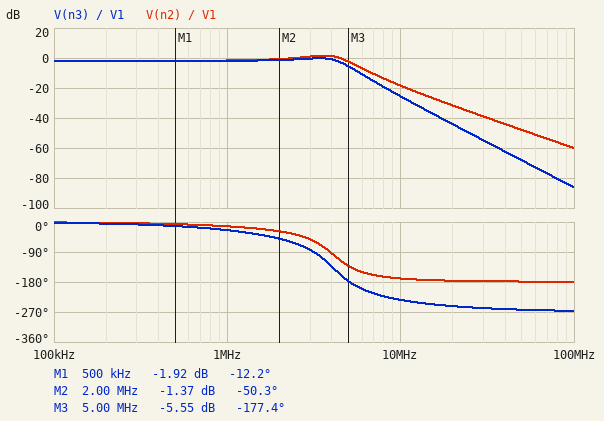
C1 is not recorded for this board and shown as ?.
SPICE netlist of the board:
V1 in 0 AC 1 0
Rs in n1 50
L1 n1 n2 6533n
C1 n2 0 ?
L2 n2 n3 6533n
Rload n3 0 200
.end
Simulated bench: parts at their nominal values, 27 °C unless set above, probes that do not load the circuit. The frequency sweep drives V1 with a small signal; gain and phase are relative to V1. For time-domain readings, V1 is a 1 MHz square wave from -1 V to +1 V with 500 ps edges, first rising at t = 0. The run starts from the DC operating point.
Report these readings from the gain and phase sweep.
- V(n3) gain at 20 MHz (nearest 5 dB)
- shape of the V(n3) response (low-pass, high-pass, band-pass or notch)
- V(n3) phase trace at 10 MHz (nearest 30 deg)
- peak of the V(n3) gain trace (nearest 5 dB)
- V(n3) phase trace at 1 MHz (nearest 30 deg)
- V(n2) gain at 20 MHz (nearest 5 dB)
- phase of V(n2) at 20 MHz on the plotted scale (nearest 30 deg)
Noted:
-45 dB
low-pass
-240 deg
0 dB
-30 deg
-30 dB
-180 deg
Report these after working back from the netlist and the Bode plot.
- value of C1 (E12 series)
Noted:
390 pF
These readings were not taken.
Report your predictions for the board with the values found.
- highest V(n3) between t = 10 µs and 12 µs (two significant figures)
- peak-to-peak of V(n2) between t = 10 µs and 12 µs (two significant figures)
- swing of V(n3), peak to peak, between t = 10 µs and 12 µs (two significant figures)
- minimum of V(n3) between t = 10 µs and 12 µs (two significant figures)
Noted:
1.1 V
2.5 V
2.2 V
-1.1 V
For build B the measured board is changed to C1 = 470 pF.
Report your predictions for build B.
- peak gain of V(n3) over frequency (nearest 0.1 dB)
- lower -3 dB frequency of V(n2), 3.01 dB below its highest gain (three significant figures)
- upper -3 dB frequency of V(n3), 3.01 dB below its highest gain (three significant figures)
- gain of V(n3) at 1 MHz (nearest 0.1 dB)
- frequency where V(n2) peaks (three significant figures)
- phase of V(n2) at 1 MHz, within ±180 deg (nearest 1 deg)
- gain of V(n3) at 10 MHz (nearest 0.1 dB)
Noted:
-0.1 dB
948 kHz
4.11 MHz
-1.7 dB
3.21 MHz
-14 deg
-27.5 dB
